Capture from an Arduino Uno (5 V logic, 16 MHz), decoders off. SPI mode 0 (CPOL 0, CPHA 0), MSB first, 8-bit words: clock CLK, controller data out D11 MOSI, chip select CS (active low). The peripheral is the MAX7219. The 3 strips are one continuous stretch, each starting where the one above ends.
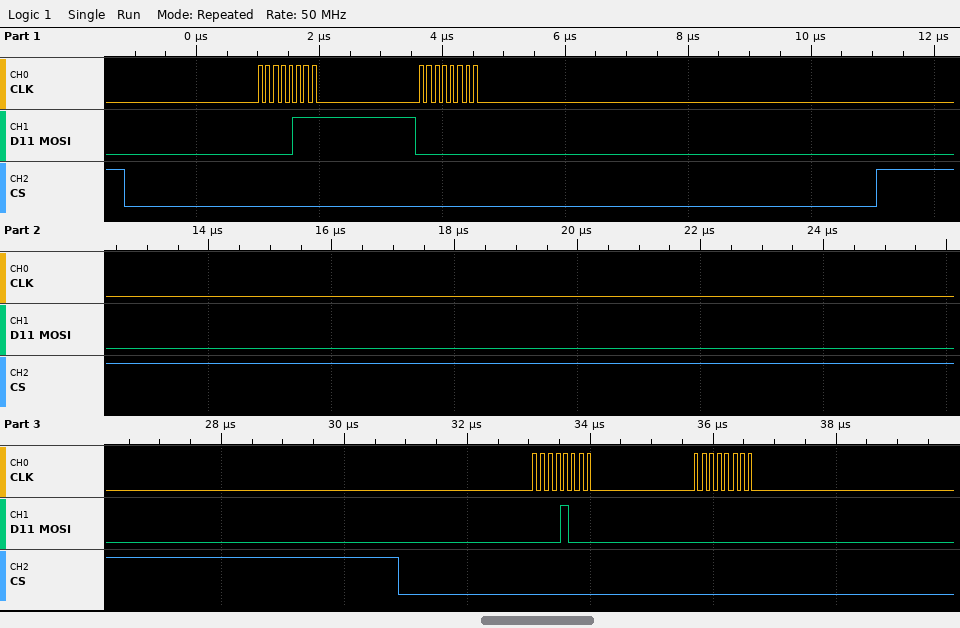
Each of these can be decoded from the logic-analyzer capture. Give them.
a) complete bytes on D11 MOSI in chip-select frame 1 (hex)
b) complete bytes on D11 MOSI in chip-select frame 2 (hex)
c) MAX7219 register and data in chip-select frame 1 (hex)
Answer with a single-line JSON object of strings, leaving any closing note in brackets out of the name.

{"complete bytes on D11 MOSI in chip-select frame 1": "07 00", "complete bytes on D11 MOSI in chip-select frame 2": "08 00", "MAX7219 register and data in chip-select frame 1": "register 0x7, data 0x00"}
